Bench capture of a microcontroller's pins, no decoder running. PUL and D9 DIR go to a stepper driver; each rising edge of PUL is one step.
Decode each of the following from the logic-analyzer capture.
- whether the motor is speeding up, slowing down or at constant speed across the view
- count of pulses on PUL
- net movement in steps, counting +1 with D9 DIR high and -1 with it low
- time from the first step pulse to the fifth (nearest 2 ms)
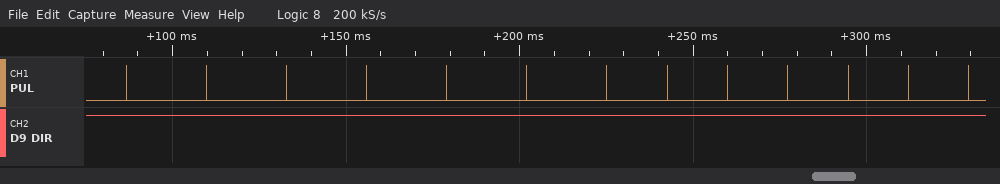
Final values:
speeding up
13
+13
92 ms
